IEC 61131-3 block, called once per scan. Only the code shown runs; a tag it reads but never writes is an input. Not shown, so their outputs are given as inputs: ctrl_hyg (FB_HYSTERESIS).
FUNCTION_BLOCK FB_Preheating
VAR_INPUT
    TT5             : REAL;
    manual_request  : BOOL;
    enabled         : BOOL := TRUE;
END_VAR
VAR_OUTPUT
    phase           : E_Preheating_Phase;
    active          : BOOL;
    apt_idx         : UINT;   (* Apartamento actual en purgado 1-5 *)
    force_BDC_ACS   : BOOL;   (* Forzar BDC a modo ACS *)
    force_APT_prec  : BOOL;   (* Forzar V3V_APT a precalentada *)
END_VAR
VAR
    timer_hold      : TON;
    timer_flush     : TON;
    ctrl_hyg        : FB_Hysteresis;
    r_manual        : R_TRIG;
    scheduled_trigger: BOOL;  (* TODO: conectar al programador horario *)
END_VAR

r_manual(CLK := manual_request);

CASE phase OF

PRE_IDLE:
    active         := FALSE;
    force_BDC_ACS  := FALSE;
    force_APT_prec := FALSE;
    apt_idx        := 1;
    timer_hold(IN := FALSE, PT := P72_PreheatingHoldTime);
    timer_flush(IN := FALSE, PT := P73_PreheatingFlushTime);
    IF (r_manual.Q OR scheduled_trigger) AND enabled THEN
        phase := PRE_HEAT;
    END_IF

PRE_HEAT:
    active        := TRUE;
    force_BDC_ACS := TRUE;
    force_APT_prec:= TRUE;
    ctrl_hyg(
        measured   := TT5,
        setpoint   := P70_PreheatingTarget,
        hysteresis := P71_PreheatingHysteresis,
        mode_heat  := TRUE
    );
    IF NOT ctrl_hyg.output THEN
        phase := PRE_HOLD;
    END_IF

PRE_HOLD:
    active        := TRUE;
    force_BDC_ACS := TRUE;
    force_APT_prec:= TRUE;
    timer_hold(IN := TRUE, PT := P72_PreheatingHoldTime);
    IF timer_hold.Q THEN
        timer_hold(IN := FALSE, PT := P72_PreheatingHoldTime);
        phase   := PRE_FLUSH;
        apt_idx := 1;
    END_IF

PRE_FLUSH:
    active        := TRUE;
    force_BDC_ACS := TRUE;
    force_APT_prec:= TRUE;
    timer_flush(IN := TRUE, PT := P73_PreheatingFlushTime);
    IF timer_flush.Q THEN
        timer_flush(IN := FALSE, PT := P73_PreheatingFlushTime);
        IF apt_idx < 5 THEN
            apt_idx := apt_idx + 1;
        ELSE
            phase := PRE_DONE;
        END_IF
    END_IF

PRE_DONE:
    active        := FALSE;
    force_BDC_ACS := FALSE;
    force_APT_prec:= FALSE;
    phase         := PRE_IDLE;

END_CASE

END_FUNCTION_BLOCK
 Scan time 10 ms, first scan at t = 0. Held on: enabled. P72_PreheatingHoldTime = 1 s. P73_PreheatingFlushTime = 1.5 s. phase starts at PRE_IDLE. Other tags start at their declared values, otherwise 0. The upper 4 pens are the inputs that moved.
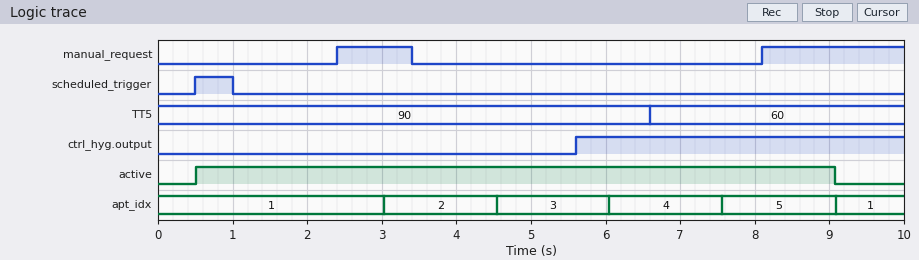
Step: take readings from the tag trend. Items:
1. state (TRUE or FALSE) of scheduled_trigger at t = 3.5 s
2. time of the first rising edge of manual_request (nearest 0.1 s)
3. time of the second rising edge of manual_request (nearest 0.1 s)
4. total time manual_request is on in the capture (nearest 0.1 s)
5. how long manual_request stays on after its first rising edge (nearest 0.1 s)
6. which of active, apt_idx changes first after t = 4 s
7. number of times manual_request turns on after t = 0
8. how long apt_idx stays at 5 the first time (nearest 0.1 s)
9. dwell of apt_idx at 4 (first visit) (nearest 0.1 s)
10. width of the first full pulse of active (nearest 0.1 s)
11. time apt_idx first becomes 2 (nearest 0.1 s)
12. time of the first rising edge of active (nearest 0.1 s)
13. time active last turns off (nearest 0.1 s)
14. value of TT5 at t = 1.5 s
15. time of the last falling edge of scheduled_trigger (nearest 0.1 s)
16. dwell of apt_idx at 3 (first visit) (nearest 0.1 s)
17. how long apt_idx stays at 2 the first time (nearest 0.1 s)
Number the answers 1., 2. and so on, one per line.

1. FALSE
2. 2.4 s
3. 8.1 s
4. 2.9 s
5. 1.0 s
6. apt_idx
7. 2
8. 1.5 s
9. 1.5 s
10. 8.6 s
11. 3.0 s
12. 0.5 s
13. 9.1 s
14. 90
15. 1.0 s
16. 1.5 s
17. 1.5 s
